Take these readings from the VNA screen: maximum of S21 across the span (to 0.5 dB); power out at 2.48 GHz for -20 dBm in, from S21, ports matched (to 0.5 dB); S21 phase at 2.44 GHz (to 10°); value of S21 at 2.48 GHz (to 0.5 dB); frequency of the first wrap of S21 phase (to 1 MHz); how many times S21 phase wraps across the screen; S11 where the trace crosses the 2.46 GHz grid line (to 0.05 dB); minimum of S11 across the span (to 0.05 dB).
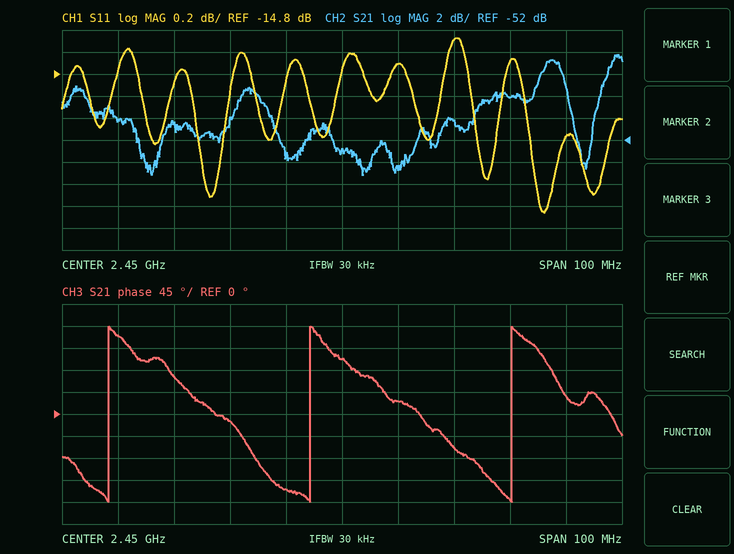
-44.0 dB
-68.0 dBm
-150°
-48.0 dB
2.408 GHz
3
-14.70 dB
-16.05 dB
